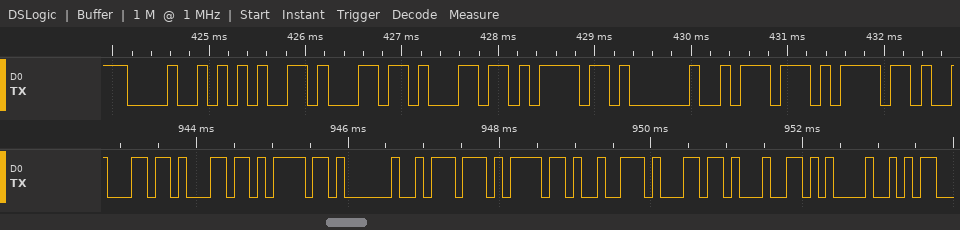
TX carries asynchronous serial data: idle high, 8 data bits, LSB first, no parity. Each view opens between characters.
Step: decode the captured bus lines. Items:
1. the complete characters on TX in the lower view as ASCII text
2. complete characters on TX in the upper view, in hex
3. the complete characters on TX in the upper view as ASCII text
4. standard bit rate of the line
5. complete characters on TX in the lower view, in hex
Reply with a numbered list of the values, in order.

1. "llo world!"
2. 48, 65, 6C, 6C, 6F, 20, 77, 6F
3. "Hello wo"
4. 9600 baud
5. 6C, 6C, 6F, 20, 77, 6F, 72, 6C, 64, 21
